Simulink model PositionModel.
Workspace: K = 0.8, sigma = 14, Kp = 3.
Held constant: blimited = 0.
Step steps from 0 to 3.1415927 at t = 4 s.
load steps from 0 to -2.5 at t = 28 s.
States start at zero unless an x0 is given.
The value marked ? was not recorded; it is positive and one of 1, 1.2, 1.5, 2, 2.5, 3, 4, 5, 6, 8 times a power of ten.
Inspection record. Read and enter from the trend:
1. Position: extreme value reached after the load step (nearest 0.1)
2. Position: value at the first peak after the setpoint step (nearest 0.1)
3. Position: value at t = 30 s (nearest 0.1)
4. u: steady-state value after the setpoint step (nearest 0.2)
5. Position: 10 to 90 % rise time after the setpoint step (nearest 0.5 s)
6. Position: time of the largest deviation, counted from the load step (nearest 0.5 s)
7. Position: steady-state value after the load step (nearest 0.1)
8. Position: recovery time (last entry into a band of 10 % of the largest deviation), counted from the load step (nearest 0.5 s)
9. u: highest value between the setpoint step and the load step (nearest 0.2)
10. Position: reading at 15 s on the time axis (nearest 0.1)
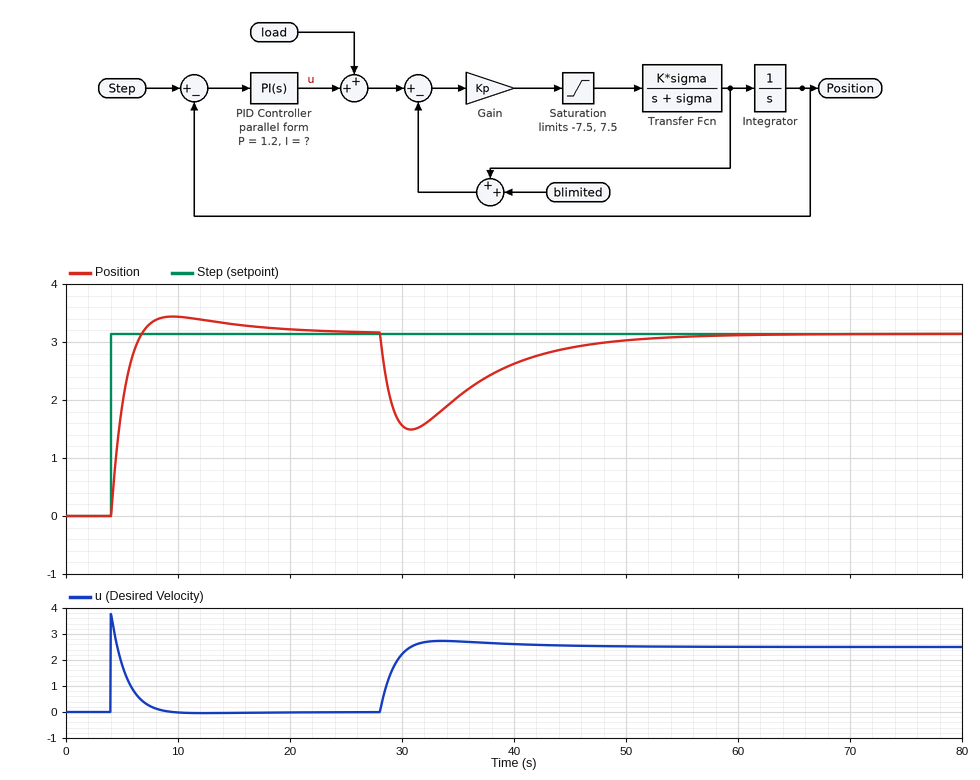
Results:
1.5
3.4
1.6
0.0
2.0 s
3.0 s
3.1
19.5 s
3.8
3.3
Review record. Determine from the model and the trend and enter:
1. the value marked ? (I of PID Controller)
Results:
0.15
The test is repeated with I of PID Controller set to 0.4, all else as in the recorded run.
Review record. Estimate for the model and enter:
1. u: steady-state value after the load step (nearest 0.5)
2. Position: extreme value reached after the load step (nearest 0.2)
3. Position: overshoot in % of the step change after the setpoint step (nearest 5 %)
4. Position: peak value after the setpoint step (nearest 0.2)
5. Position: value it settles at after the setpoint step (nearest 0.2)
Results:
2.5
1.8
20 %
3.8
3.2
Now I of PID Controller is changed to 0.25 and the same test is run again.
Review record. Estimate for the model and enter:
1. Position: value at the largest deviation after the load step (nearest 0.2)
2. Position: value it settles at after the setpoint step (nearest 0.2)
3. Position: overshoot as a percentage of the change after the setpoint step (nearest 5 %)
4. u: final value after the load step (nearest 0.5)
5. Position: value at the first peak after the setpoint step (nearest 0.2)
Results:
1.6
3.2
15 %
2.5
3.6
